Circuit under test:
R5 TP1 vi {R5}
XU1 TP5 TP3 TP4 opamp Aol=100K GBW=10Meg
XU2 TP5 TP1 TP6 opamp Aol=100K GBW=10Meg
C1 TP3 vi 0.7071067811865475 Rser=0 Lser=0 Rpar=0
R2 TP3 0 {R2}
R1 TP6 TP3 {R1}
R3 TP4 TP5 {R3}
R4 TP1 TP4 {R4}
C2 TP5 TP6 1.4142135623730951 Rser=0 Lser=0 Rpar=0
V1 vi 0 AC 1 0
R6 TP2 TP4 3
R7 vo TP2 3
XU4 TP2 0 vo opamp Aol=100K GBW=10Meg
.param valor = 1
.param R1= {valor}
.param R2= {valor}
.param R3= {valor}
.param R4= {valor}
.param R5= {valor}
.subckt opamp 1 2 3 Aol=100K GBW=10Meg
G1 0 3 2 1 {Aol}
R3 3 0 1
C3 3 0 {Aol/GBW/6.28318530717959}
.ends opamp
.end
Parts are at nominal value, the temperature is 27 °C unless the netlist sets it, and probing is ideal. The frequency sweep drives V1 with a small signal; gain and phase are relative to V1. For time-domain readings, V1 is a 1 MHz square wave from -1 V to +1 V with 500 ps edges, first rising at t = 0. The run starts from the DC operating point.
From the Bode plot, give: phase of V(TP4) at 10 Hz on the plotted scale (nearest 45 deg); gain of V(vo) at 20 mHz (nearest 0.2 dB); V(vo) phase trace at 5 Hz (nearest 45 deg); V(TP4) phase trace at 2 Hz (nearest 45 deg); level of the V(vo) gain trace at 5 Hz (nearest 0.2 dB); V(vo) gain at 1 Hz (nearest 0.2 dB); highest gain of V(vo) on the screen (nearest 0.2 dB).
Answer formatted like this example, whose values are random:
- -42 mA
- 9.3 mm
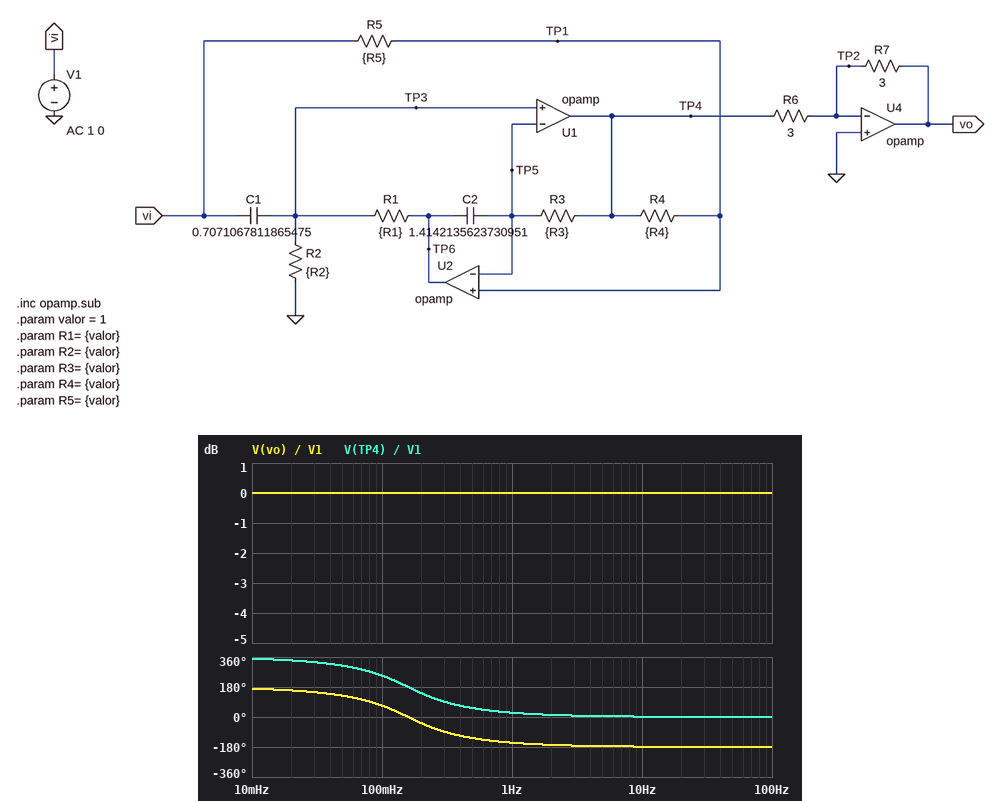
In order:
- 0 deg
- 0 dB
- -180 deg
- 0 deg
- 0 dB
- 0 dB
- 0 dB
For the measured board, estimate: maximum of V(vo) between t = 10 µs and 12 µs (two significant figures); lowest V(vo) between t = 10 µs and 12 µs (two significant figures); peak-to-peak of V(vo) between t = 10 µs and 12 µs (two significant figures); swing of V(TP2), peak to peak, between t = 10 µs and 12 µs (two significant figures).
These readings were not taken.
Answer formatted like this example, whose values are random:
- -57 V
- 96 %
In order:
- 1.1 V
- -1.1 V
- 2.2 V
- 1.3 V
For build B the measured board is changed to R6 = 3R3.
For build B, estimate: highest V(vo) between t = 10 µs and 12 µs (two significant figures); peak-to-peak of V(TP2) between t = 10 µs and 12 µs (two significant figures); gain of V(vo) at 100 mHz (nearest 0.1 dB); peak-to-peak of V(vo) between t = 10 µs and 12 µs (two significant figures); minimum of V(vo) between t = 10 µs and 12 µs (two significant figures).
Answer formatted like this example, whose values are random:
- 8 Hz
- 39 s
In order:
- 1.0 V
- 1.2 V
- -0.8 dB
- 2.0 V
- -1.0 V
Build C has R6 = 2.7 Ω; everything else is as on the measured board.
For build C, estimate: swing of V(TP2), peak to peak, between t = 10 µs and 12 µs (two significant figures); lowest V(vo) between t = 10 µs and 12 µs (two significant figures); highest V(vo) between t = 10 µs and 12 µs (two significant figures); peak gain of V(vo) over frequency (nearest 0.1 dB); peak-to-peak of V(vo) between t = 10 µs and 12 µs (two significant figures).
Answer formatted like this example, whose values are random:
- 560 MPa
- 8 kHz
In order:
- 1.4 V
- -1.2 V
- 1.2 V
- 0.9 dB
- 2.4 V
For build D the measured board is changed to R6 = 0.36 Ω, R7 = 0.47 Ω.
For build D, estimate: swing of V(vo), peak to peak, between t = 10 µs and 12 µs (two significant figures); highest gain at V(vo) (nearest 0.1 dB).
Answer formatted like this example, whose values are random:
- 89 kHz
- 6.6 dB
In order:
- 2.7 V
- 2.3 dB
